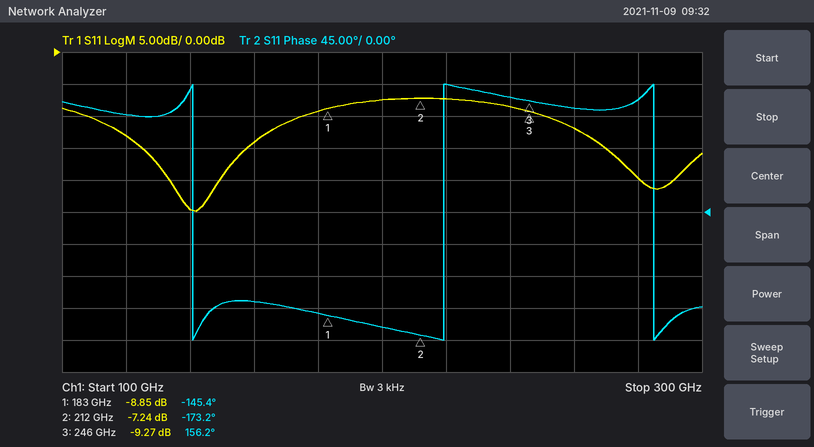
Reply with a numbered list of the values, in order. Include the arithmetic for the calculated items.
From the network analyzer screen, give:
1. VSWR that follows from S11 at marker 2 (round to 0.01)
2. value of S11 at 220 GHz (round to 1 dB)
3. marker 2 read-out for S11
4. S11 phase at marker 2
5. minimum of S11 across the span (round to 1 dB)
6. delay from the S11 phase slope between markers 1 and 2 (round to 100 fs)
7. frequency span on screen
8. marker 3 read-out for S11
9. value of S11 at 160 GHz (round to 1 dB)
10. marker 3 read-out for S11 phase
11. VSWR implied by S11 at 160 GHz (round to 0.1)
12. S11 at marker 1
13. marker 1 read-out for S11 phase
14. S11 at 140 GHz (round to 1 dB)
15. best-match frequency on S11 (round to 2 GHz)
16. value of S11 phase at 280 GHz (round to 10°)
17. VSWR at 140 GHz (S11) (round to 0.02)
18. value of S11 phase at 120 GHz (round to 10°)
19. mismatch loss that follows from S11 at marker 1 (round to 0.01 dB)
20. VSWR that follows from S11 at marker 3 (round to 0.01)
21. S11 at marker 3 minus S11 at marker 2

1. (1 + 0.4345)/(1 − 0.4345) ≈ 2.54
2. -7 dB
3. -7.24 dB
4. -173.2°
5. -25 dB
6. −(-173.2° − (-145.4°))/(360° × 29 GHz) ≈ 2.7 ps
7. 200 GHz
8. -9.27 dB
9. -14 dB
10. 156.2°
11. |Γ| = 10^(-14/20) = 0.1995; VSWR = (1 + 0.1995)/(1 − 0.1995) ≈ 1.5
12. -8.85 dB
13. -145.4°
14. -25 dB
15. 142 GHz
16. 160°
17. |Γ| = 10^(-25/20) = 0.0562; VSWR = (1 + 0.0562)/(1 − 0.0562) ≈ 1.12
18. 140°
19. −10 log10(1 − 10^(-8.85/10)) ≈ 0.61 dB
20. (1 + 0.3440)/(1 − 0.3440) ≈ 2.05
21. -9.27 − (-7.24) = -2.03 dB
